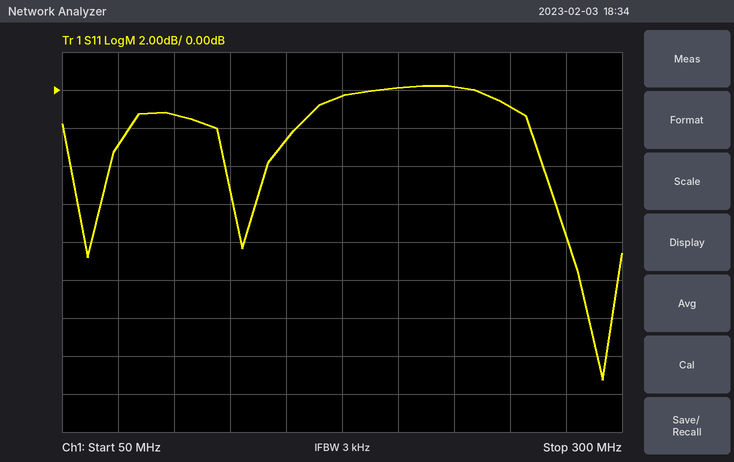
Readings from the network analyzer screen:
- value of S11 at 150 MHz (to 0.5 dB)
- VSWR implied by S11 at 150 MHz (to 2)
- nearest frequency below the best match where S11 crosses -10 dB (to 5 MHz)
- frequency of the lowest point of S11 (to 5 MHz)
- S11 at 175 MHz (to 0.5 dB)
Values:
-2.5 dB
6
280 MHz
290 MHz
-0.5 dB
